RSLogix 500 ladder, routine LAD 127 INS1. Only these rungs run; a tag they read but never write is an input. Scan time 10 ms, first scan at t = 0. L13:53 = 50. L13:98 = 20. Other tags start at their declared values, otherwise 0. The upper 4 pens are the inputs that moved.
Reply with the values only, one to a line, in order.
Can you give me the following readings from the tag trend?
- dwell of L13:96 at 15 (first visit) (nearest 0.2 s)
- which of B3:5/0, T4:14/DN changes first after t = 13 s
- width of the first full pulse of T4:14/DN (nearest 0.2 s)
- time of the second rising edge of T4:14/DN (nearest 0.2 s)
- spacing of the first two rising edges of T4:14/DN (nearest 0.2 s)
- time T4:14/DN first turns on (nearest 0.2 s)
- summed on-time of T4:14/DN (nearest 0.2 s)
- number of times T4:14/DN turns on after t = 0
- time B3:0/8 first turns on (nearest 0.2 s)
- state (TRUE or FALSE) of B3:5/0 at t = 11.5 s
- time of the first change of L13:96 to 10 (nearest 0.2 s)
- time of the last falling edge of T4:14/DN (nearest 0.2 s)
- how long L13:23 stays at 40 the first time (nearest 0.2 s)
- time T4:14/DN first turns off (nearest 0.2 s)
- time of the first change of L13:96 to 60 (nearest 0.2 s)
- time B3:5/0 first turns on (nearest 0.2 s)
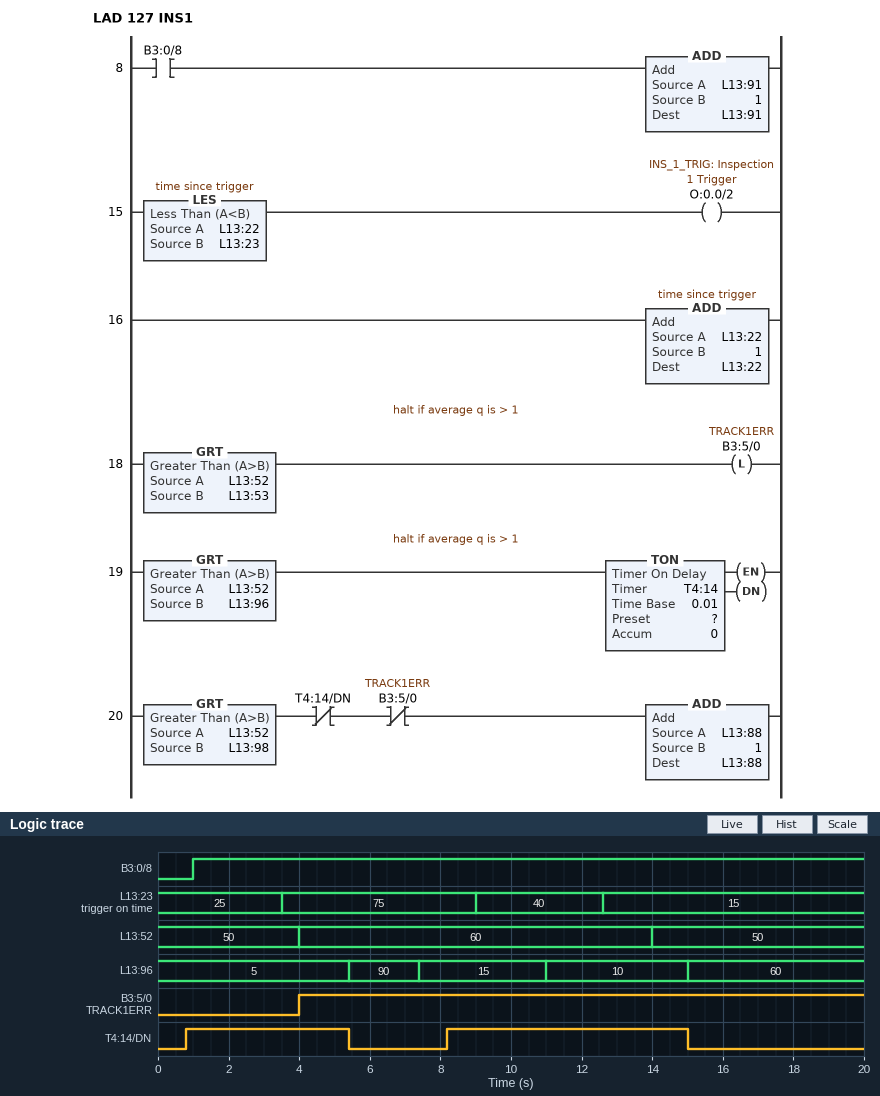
3.6 s
T4:14/DN
4.6 s
8.2 s
7.4 s
0.8 s
11.4 s
2
1.0 s
TRUE
11.0 s
15.0 s
3.6 s
5.4 s
15.0 s
4.0 s
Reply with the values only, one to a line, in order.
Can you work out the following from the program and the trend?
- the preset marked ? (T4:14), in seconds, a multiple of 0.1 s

0.8 s
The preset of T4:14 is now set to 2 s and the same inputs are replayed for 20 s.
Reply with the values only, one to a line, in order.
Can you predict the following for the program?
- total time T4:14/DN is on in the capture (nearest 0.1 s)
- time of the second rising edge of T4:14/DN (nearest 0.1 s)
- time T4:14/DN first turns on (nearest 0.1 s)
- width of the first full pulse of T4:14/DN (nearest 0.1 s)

9.0 s
9.4 s
2.0 s
3.4 s
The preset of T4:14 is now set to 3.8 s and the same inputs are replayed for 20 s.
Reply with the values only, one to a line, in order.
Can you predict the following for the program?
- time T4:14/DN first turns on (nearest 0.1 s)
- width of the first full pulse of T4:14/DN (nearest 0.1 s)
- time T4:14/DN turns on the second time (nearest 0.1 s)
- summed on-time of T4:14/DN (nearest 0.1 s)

3.8 s
1.6 s
11.2 s
5.4 s
